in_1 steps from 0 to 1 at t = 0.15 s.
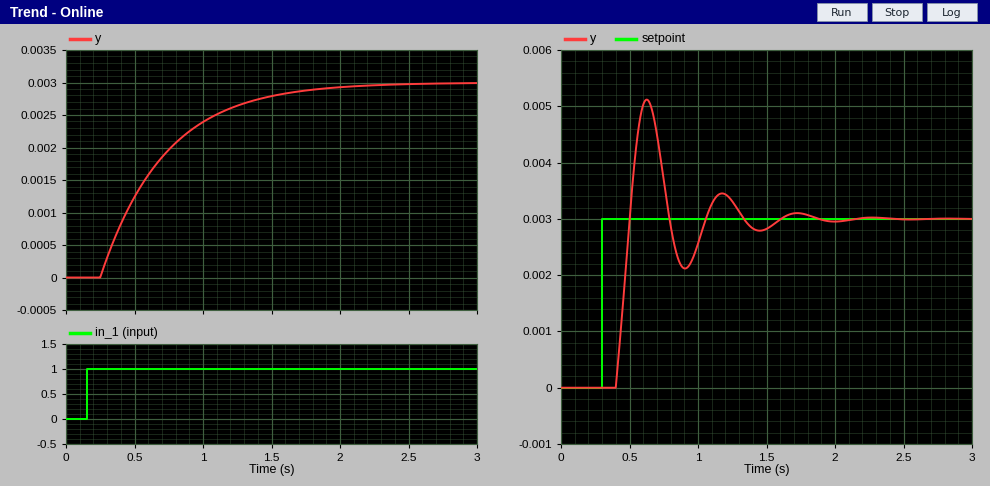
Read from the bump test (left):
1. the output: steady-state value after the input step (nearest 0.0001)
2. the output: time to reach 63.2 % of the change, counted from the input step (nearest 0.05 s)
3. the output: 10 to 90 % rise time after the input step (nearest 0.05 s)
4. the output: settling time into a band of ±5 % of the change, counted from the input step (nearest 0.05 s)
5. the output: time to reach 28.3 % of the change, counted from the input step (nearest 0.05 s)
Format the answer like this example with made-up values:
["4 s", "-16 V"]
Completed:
["0.0030", "0.55 s", "1.05 s", "1.50 s", "0.25 s"]
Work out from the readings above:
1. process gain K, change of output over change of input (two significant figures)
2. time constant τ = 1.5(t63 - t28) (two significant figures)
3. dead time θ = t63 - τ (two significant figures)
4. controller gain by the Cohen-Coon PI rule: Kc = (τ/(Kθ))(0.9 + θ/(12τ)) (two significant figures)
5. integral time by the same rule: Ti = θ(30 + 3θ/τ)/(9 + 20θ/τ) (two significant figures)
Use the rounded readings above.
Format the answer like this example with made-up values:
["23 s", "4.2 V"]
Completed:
["0.0030", "0.45 s", "0.10 s", "1400", "0.23 s"]
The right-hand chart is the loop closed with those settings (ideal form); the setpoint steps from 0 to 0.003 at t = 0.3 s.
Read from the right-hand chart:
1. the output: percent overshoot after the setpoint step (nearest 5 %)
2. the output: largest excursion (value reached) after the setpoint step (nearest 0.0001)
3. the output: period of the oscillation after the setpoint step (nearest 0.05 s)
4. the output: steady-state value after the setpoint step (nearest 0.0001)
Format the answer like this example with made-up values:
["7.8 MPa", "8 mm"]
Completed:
["70 %", "0.0051", "0.55 s", "0.0030"]
